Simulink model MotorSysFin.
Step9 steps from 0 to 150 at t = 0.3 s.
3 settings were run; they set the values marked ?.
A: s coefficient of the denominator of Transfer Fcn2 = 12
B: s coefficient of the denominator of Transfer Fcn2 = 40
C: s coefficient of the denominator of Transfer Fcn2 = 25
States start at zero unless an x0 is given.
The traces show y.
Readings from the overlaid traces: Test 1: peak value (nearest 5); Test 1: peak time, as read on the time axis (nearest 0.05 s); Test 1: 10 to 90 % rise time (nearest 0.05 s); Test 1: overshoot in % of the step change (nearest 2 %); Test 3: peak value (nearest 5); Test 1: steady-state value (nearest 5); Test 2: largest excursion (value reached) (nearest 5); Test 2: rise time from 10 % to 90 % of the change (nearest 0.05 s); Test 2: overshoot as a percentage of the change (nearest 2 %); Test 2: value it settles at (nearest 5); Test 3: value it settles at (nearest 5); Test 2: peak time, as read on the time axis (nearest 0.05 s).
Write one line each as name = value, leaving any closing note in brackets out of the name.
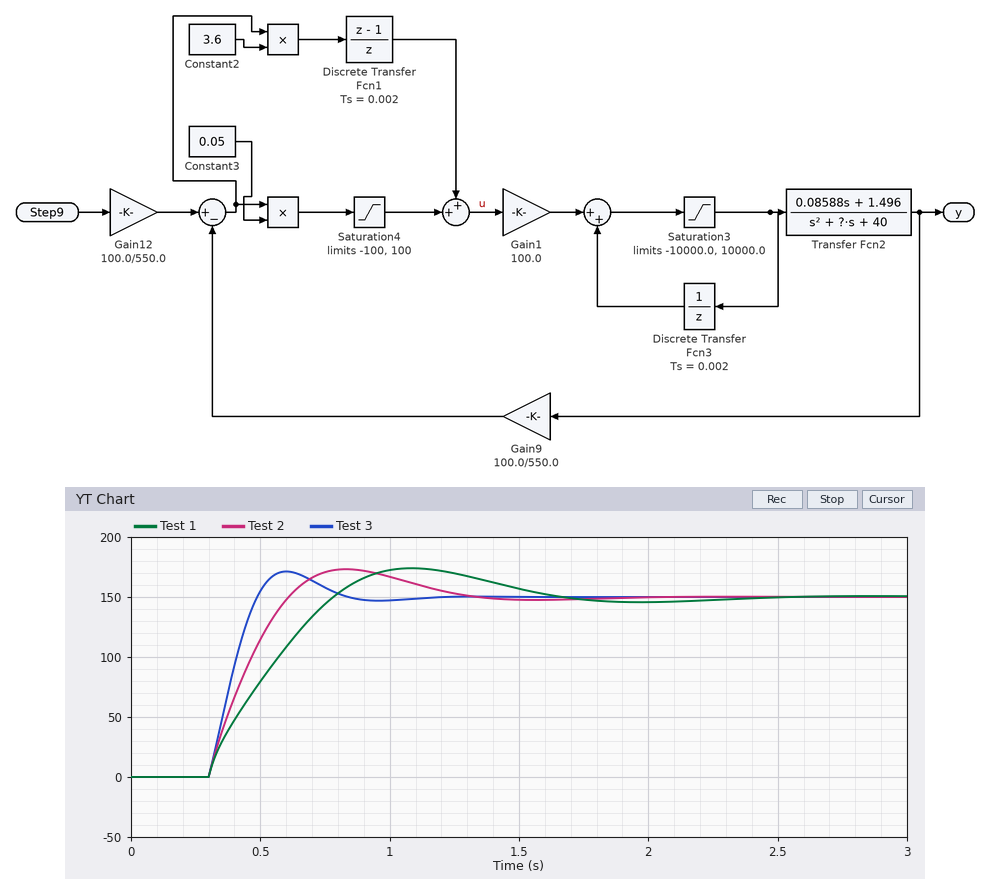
Test 1: peak value = 175
Test 1: peak time, as read on the time axis = 1.10 s
Test 1: 10 to 90 % rise time = 0.40 s
Test 1: overshoot in % of the step change = 16 %
Test 3: peak value = 170
Test 1: steady-state value = 150
Test 2: largest excursion (value reached) = 175
Test 2: rise time from 10 % to 90 % of the change = 0.25 s
Test 2: overshoot as a percentage of the change = 16 %
Test 2: value it settles at = 150
Test 3: value it settles at = 150
Test 2: peak time, as read on the time axis = 0.85 s
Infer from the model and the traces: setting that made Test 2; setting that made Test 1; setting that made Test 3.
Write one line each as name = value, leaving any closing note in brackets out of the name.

setting that made Test 2 = C
setting that made Test 1 = B
setting that made Test 3 = A
